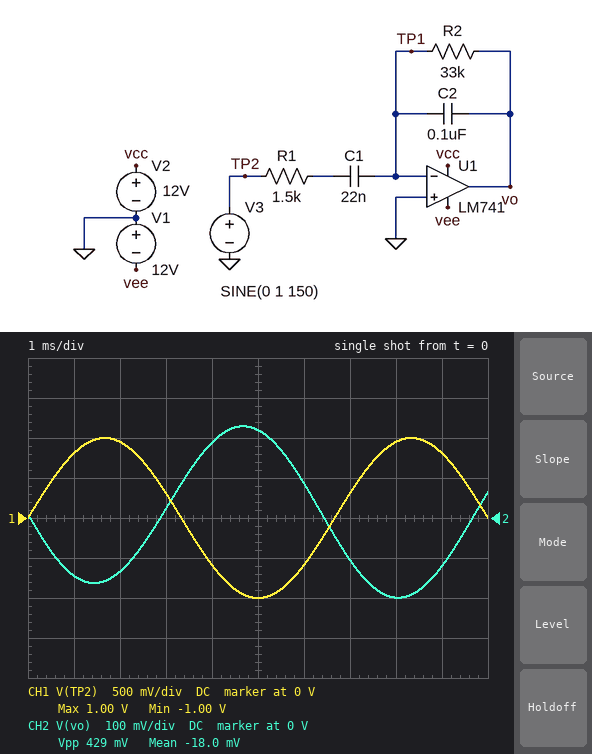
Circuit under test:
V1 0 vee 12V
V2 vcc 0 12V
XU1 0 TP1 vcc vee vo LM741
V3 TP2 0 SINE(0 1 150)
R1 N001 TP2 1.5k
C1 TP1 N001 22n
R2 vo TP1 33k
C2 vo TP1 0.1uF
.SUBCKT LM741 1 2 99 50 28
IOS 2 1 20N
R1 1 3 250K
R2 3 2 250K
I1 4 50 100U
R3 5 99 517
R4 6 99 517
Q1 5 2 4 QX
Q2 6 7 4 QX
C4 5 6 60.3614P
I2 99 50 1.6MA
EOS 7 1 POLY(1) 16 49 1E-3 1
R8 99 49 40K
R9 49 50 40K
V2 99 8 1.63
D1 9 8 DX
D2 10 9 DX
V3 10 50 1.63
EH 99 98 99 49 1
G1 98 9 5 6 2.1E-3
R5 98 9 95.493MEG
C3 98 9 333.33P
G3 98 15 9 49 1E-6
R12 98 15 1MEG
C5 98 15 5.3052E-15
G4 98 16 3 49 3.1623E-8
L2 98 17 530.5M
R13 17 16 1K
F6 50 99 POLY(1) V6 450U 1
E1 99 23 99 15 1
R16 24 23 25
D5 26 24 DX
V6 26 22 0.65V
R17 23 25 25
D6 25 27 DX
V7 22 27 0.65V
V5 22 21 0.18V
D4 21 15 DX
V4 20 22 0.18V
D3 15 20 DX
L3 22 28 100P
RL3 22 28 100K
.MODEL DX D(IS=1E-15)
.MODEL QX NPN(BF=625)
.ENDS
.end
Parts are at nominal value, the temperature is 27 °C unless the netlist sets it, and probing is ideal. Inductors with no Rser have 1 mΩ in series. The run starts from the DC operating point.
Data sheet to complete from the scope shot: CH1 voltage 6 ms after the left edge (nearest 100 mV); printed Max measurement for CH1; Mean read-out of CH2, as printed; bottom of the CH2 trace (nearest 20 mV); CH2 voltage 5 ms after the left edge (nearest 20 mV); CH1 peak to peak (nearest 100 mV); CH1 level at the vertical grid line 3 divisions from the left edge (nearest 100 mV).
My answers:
-600 mV
1.00 V
-18.0 mV
-200 mV
220 mV
2.0 V
300 mV
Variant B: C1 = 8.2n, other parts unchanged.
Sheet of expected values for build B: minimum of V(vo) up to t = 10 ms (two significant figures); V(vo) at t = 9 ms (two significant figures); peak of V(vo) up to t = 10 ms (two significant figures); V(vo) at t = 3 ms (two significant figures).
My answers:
-72 mV
-41 mV
88 mV
13 mV
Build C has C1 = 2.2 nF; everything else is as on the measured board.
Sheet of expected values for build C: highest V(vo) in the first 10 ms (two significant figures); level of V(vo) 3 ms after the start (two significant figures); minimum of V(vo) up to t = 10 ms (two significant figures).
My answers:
27 mV
6.8 mV
-16 mV
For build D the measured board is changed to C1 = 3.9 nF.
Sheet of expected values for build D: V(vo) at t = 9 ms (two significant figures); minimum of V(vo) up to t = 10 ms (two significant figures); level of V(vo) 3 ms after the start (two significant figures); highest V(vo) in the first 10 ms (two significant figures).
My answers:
-17 mV
-32 mV
8.6 mV
44 mV
